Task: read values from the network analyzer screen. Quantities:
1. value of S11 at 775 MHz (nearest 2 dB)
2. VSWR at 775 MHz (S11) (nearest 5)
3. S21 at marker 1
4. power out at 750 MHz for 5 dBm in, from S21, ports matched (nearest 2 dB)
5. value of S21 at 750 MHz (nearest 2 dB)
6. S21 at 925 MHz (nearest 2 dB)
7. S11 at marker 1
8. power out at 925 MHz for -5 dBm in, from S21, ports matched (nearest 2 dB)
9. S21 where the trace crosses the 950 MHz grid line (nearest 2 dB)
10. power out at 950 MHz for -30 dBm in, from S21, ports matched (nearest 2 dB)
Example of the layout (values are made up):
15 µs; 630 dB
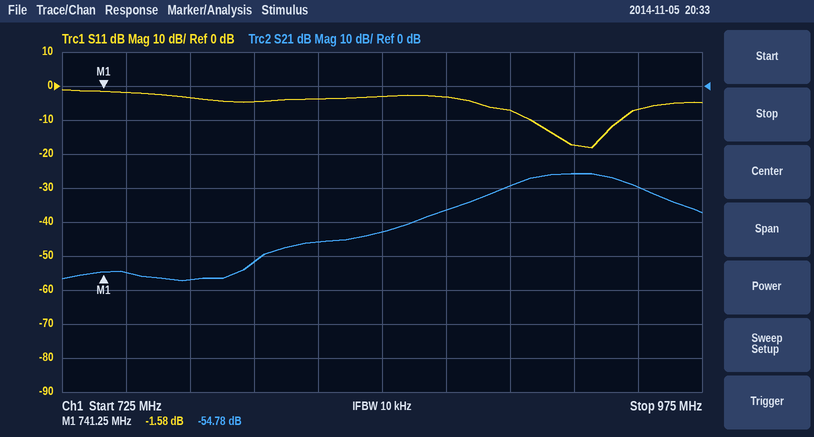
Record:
-4 dB; 5; -54.78 dB; -50 dBm; -54 dB; -26 dB; -1.58 dB; -30 dBm; -30 dB; -60 dBm
